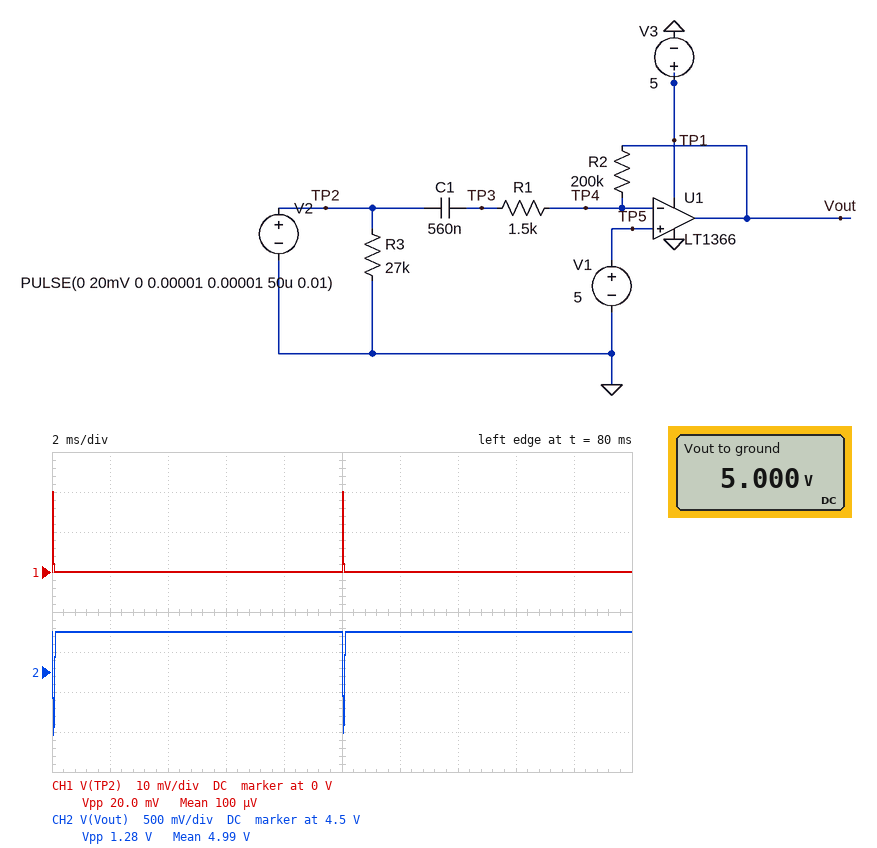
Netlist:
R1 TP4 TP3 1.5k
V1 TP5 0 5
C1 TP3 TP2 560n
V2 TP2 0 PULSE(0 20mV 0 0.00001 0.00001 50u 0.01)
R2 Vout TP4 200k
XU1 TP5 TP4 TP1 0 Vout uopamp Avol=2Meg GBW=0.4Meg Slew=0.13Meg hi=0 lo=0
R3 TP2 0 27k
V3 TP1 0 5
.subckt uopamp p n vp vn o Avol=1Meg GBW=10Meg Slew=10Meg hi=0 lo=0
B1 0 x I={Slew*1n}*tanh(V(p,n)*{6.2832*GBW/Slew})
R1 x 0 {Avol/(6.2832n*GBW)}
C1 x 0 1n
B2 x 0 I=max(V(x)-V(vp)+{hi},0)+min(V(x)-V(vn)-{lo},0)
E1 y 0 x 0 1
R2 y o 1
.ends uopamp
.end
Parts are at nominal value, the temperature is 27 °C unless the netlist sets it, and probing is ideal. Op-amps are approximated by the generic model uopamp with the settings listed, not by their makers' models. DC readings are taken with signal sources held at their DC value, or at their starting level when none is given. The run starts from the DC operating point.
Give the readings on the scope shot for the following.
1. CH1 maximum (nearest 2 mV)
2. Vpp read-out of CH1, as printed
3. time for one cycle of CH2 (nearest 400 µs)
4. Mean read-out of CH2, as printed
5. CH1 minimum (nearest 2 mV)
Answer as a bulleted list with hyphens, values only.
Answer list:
- 20 mV
- 20.0 mV
- 10.0 ms
- 4.99 V
- 0 V
